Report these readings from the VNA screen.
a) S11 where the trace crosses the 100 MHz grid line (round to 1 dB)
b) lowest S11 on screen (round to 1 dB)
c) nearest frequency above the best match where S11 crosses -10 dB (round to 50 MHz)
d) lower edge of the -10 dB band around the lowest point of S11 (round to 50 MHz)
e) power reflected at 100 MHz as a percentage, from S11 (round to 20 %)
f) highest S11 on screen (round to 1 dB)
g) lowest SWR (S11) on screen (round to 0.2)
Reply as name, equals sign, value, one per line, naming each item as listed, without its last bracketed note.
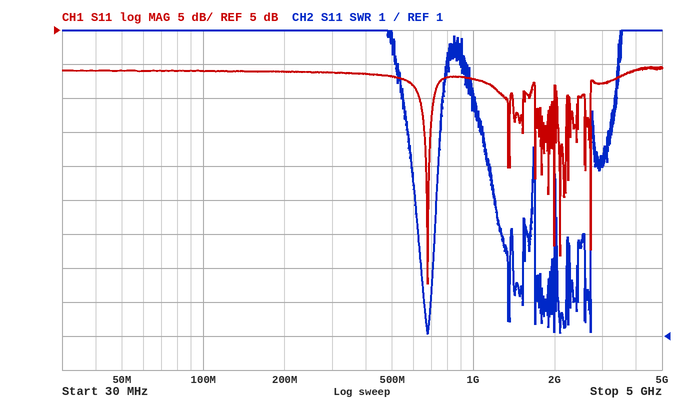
S11 where the trace crosses the 100 MHz grid line = -1 dB
lowest S11 on screen = -32 dB
nearest frequency above the best match where S11 crosses -10 dB = 700 MHz
lower edge of the -10 dB band around the lowest point of S11 = 650 MHz
power reflected at 100 MHz as a percentage, from S11 = 80 %
highest S11 on screen = 0 dB
lowest SWR (S11) on screen = 1.0
